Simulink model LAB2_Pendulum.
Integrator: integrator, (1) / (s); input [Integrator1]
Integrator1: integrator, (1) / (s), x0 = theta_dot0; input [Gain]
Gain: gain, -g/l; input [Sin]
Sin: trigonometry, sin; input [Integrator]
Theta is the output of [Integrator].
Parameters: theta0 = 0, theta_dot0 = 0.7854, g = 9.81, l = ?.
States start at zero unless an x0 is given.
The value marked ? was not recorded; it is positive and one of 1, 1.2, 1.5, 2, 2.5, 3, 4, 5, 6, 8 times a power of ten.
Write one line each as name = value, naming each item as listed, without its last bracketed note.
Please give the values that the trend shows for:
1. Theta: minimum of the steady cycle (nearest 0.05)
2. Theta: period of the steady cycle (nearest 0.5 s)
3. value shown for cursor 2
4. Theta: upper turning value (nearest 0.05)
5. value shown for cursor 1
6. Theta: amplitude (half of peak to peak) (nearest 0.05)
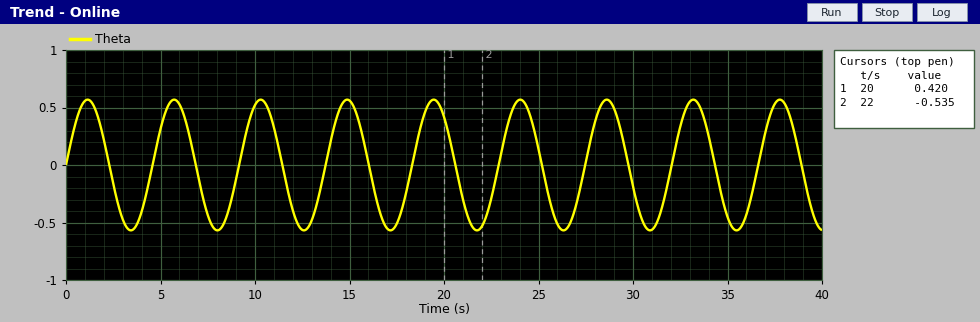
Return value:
Theta: minimum of the steady cycle = -0.55
Theta: period of the steady cycle = 4.5 s
value shown for cursor 2 = -0.535
Theta: upper turning value = 0.55
value shown for cursor 1 = 0.420
Theta: amplitude (half of peak to peak) = 0.55
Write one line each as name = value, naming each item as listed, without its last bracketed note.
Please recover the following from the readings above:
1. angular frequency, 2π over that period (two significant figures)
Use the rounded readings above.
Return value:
angular frequency, 2π over that period = 1.4 rad/s
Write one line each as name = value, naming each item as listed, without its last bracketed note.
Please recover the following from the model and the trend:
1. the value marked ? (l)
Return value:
the value marked ? = 5
